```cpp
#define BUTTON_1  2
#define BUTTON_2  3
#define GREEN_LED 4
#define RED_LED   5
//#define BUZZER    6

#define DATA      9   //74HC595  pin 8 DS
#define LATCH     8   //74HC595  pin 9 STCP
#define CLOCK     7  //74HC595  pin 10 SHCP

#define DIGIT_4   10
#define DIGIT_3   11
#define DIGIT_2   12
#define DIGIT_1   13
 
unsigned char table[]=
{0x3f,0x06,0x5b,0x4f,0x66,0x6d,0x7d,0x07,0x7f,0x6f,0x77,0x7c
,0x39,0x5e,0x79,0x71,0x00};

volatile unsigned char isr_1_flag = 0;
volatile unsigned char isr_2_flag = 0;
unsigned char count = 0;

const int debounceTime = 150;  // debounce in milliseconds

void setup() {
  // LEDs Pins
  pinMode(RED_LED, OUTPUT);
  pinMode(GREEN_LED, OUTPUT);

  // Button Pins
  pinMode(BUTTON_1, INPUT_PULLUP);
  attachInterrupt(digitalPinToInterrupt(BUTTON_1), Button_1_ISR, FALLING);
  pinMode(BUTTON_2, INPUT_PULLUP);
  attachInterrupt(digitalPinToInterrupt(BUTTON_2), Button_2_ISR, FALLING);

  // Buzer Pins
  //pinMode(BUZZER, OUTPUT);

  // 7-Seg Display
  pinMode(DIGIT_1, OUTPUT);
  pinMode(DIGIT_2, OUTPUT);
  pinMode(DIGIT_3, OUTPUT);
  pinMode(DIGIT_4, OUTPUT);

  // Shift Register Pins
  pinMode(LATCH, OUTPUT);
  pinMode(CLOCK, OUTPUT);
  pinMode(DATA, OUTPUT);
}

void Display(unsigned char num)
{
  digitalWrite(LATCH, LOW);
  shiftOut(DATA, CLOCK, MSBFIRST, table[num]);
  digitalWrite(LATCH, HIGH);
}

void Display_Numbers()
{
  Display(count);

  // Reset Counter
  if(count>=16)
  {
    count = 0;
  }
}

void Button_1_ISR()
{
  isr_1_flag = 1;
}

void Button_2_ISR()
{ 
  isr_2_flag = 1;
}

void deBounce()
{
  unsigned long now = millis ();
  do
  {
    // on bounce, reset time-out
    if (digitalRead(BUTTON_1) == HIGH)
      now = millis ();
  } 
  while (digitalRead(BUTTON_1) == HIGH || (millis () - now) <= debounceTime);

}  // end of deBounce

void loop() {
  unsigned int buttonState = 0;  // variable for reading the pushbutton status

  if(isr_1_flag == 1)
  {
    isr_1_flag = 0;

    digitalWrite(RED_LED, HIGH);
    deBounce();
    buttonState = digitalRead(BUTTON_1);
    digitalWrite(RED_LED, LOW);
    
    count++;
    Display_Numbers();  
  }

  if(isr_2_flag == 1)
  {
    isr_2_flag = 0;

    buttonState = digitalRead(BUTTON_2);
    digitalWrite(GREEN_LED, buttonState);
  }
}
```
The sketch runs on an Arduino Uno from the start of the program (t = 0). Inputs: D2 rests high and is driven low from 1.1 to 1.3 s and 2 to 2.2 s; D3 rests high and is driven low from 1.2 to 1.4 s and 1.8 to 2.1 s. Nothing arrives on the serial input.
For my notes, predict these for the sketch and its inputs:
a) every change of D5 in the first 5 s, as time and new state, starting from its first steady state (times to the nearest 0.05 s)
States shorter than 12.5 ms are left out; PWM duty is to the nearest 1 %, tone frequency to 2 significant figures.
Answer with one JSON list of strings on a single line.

["0 s low; 1.1 s high; 1.25 s low; 2 s high; 2.15 s low"]
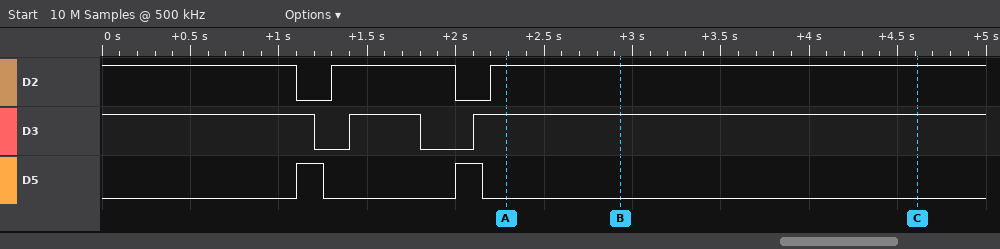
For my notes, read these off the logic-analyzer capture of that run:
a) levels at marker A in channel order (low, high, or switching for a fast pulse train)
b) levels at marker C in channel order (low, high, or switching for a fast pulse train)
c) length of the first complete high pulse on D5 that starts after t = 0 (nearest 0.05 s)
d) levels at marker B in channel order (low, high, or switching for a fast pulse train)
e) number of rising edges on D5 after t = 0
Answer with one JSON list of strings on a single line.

["D2 high, D3 high, D5 low", "D2 high, D3 high, D5 low", "0.15 s", "D2 high, D3 high, D5 low", "2"]
